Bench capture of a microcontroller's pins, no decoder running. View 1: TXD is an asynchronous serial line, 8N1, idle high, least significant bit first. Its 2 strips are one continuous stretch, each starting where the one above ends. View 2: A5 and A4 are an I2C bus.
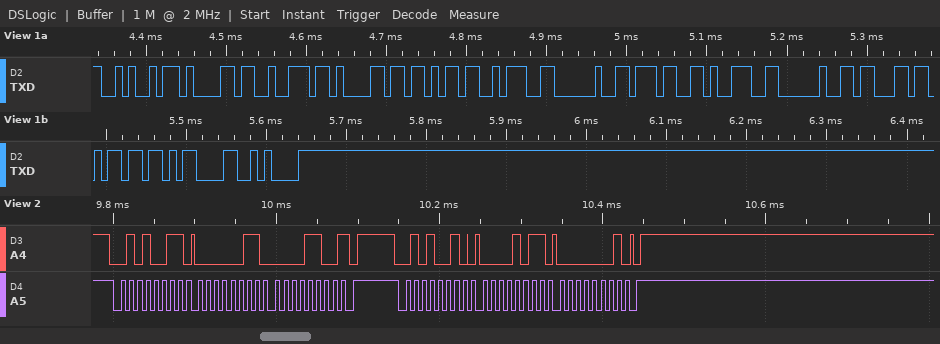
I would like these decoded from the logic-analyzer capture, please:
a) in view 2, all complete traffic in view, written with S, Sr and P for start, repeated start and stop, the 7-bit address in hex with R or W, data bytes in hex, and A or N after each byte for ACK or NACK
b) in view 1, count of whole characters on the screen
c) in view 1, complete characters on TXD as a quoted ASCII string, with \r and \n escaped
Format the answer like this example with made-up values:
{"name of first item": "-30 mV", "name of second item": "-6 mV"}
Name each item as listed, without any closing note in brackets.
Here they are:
{"in view 2, all complete traffic in view, written with S, Sr and P for start, repeated start and stop, the 7-bit address in hex with R or W, data bytes in hex, and A or N after each byte for ACK or NACK": "S 29R A 03 A 0C N P S 29W A 0B A 01 A P", "in view 1, count of whole characters on the screen": "14", "in view 1, complete characters on TXD as a quoted ASCII string, with \\r and \\n escaped": "\"Jarak: 79 cm\\r\\n\""}
